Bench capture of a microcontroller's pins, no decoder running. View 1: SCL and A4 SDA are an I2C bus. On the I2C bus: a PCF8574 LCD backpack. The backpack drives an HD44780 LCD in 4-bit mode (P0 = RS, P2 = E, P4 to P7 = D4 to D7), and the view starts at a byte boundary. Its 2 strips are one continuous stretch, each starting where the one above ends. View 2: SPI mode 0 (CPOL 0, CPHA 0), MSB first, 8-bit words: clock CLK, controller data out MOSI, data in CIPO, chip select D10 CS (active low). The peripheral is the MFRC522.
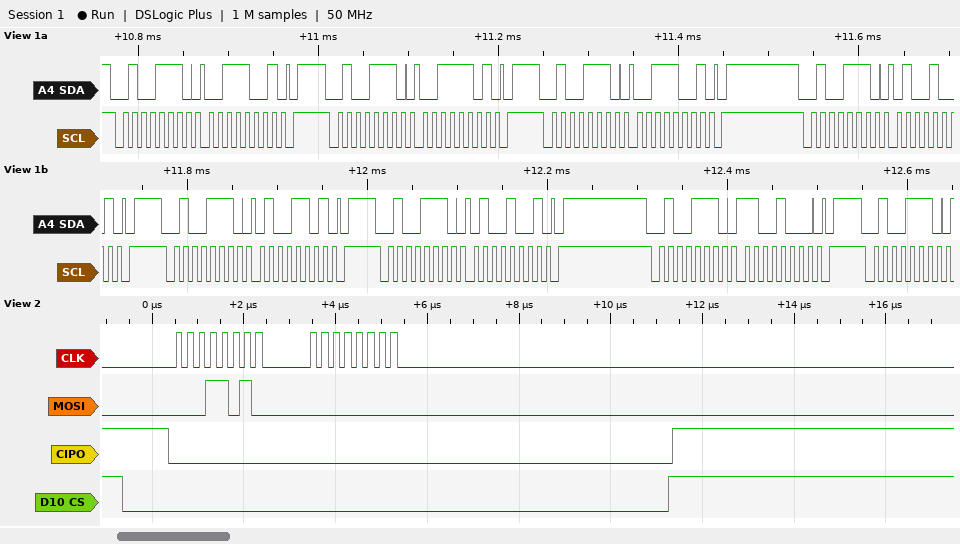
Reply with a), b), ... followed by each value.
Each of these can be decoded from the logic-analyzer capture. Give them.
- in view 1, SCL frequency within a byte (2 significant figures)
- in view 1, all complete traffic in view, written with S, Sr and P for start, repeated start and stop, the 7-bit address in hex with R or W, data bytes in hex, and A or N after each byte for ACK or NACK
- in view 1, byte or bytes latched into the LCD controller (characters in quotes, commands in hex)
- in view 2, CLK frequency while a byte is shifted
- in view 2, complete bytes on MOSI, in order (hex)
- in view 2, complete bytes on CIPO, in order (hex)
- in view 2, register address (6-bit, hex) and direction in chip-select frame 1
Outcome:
a) 100 kHz
b) S 27W A 39 A P S 27W A 3D A P S 27W A 39 A P S 27W A 49 A P S 27W A 4D A P S 27W A 49 A P S 27W A C8 A P S 27W A
c) '4'
d) 4 MHz
e) 1A 00
f) 00 00
g) 0x0D write
